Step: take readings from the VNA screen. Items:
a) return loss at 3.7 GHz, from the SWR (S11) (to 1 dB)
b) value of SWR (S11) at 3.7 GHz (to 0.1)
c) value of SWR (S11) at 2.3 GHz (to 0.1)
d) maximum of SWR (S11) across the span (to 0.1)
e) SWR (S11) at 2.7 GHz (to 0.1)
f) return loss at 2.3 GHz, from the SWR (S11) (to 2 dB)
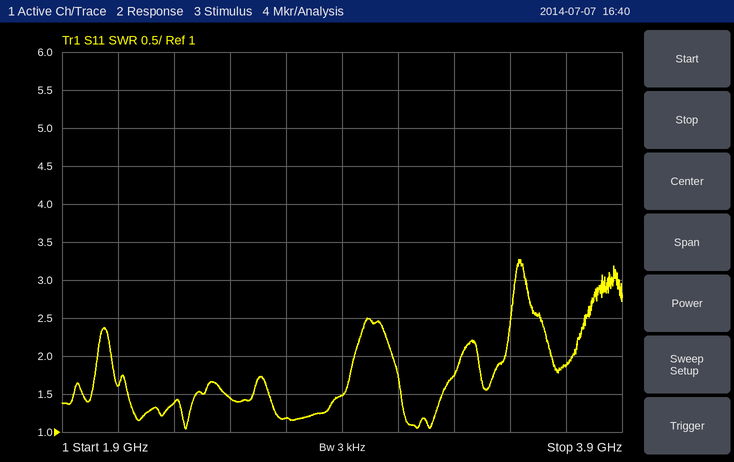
10 dB
1.9
1.4
3.3
1.2
16 dB
